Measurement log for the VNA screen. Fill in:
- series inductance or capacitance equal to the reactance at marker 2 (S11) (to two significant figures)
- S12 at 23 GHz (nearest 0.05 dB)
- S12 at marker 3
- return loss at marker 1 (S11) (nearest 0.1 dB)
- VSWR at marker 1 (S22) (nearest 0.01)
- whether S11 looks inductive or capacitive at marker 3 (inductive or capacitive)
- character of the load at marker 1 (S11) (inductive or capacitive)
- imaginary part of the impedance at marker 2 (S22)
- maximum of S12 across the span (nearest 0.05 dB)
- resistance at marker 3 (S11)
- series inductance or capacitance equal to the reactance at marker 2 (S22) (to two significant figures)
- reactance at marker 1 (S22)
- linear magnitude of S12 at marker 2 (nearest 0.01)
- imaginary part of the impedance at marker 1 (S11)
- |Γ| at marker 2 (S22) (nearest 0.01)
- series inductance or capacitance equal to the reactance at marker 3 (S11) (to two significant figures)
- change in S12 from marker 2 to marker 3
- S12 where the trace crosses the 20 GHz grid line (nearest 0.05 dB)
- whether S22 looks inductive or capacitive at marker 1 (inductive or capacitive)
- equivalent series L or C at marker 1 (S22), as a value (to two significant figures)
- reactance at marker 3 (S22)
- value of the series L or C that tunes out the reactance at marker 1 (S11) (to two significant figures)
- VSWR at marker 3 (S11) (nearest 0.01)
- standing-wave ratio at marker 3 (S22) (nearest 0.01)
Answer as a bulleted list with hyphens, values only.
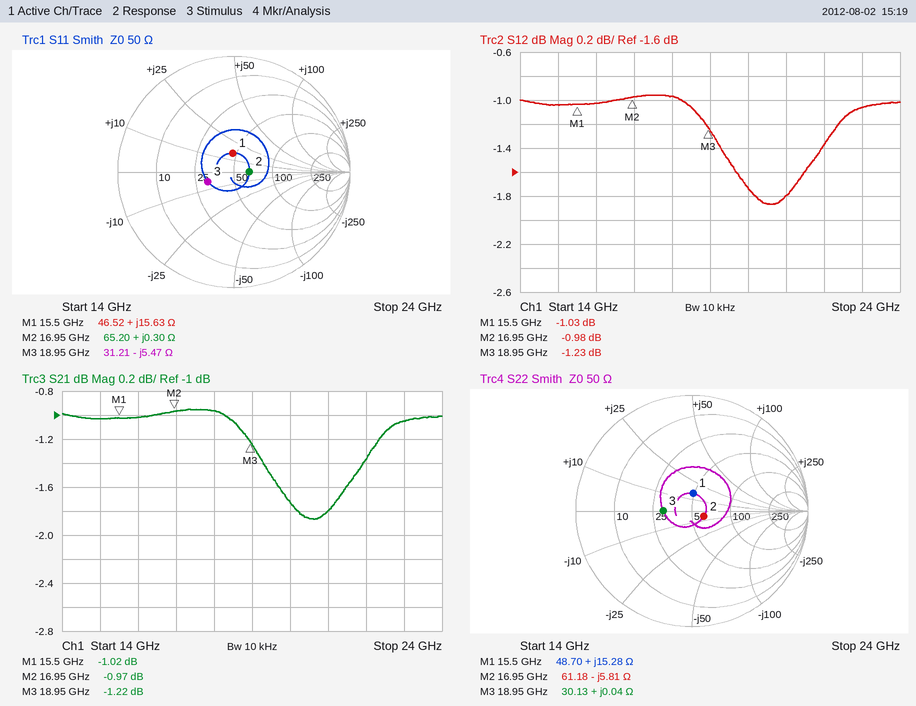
- 2.8 pH
- -1.05 dB
- -1.23 dB
- 15.7 dB
- 1.36
- capacitive
- inductive
- -5.81 Ω
- -0.95 dB
- 31.21 Ω
- 1.6 pF
- +15.28 Ω
- 0.89
- +15.63 Ω
- 0.11
- 1.5 pF
- -0.25 dB
- -1.75 dB
- inductive
- 160 pH
- +0.04 Ω
- 660 fF
- 1.63
- 1.66
